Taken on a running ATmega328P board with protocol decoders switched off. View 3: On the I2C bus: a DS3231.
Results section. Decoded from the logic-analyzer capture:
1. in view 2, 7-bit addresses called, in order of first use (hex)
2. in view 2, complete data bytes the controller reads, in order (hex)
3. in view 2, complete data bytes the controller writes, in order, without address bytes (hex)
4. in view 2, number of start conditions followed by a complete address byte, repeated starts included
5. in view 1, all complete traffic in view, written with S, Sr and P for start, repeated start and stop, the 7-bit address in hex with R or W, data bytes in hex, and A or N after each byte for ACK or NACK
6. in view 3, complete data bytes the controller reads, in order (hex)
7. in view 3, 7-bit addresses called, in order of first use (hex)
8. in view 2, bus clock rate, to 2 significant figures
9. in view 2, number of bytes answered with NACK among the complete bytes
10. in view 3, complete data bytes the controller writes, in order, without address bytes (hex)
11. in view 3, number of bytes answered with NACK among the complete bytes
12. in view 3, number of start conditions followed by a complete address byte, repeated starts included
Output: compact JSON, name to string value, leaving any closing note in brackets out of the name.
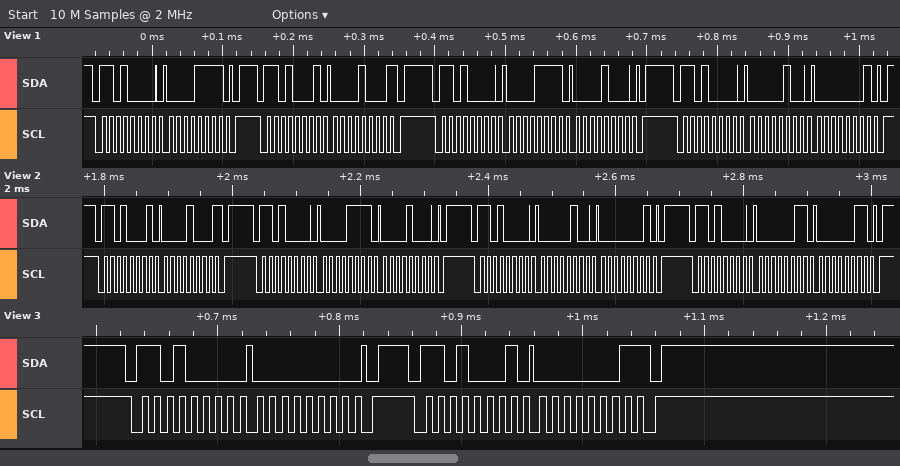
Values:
{"in view 2, 7-bit addresses called, in order of first use": "0x68", "in view 2, complete data bytes the controller reads, in order": "08", "in view 2, complete data bytes the controller writes, in order, without address bytes": "0F 08 04 01 03 03", "in view 2, number of start conditions followed by a complete address byte, repeated starts included": "4", "in view 1, all complete traffic in view, written with S, Sr and P for start, repeated start and stop, the 7-bit address in hex with R or W, data bytes in hex, and A or N after each byte for ACK or NACK": "S 68W A 0F A P S 68R A 08 N P S 68W A 0F A 08 A P S 68W A 04 A 01 A P", "in view 3, complete data bytes the controller reads, in order": "01", "in view 3, 7-bit addresses called, in order of first use": "0x68", "in view 2, bus clock rate, to 2 significant figures": "100 kHz", "in view 2, number of bytes answered with NACK among the complete bytes": "1", "in view 3, complete data bytes the controller writes, in order, without address bytes": "00", "in view 3, number of bytes answered with NACK among the complete bytes": "1", "in view 3, number of start conditions followed by a complete address byte, repeated starts included": "2"}
